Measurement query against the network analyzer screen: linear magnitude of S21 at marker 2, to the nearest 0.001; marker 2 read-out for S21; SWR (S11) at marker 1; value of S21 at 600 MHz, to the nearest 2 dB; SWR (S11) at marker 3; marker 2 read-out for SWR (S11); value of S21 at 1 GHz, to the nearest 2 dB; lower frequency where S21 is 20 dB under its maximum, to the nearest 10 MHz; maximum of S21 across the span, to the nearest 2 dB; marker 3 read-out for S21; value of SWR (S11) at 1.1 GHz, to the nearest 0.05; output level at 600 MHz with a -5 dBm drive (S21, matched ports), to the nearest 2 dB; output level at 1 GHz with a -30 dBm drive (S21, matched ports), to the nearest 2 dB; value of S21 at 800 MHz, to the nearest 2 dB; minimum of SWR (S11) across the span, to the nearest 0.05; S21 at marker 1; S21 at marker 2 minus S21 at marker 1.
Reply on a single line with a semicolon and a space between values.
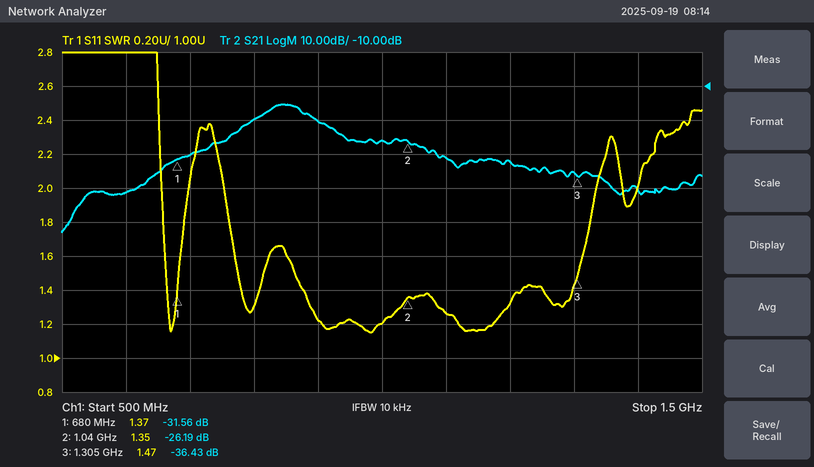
0.049; -26.19 dB; 1.37; -42 dB; 1.47; 1.35; -26 dB; 650 MHz; -16 dB; -36.43 dB; 1.25; -46 dBm; -56 dBm; -20 dB; 1.15; -31.56 dB; 5.37 dB
